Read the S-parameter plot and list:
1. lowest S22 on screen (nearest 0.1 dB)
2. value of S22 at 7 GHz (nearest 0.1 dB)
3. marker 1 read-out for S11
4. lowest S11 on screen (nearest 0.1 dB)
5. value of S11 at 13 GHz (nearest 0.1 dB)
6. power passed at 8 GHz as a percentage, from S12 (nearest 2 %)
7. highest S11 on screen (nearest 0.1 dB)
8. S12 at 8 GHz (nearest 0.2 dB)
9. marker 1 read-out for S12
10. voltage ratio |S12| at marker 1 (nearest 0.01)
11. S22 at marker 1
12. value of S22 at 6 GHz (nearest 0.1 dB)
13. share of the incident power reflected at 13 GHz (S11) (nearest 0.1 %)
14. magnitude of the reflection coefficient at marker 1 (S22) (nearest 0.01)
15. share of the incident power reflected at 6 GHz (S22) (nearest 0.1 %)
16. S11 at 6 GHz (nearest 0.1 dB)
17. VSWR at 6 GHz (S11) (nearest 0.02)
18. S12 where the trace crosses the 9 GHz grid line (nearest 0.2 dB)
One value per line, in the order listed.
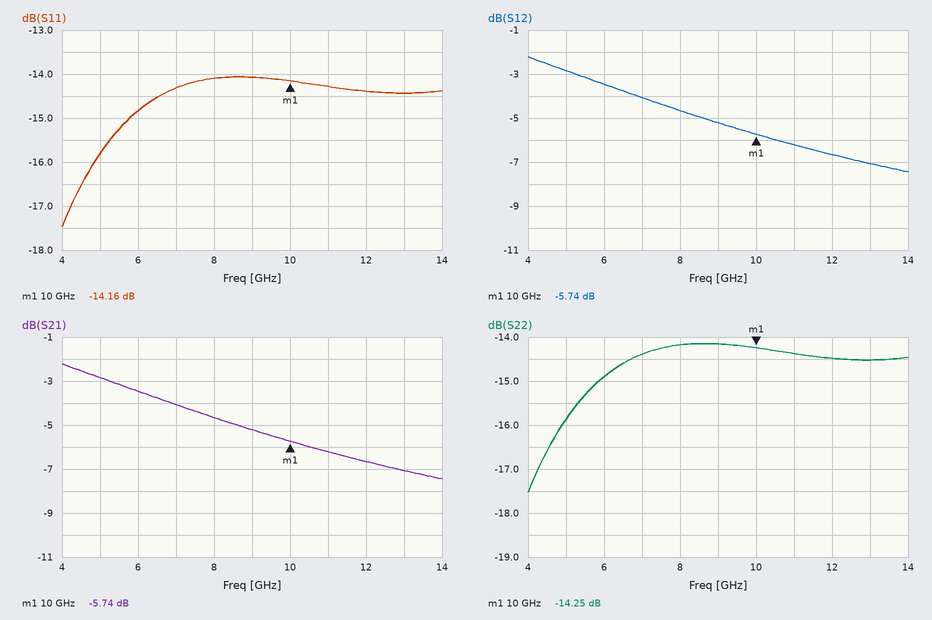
-17.5 dB
-14.4 dB
-14.16 dB
-17.5 dB
-14.4 dB
34 %
-14.1 dB
-4.6 dB
-5.74 dB
0.52
-14.25 dB
-14.9 dB
3.6 %
0.19
3.2 %
-14.8 dB
1.44
-5.2 dB
